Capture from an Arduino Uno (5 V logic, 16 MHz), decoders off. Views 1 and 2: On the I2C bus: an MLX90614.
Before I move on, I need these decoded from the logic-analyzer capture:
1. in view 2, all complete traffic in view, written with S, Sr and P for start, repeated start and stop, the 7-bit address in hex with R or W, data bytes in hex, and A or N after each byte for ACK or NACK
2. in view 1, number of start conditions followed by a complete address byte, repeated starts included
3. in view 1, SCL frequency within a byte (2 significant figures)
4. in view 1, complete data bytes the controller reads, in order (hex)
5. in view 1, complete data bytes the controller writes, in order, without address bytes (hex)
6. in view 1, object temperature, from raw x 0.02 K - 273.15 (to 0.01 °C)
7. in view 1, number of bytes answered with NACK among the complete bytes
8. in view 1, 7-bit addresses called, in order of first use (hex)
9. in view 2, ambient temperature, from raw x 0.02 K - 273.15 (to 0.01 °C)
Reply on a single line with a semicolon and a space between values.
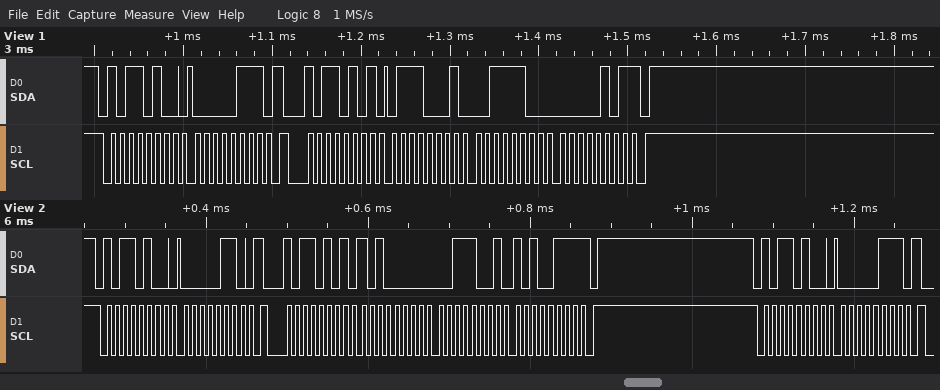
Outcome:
S 5AW A 06 A Sr 5AR A A0 A 39 A A7 N P S 5AW A 07 A; 2; 100 kHz; 71 3C 05; 07; 36.31 °C; 1; 0x5A; 21.89 °C
